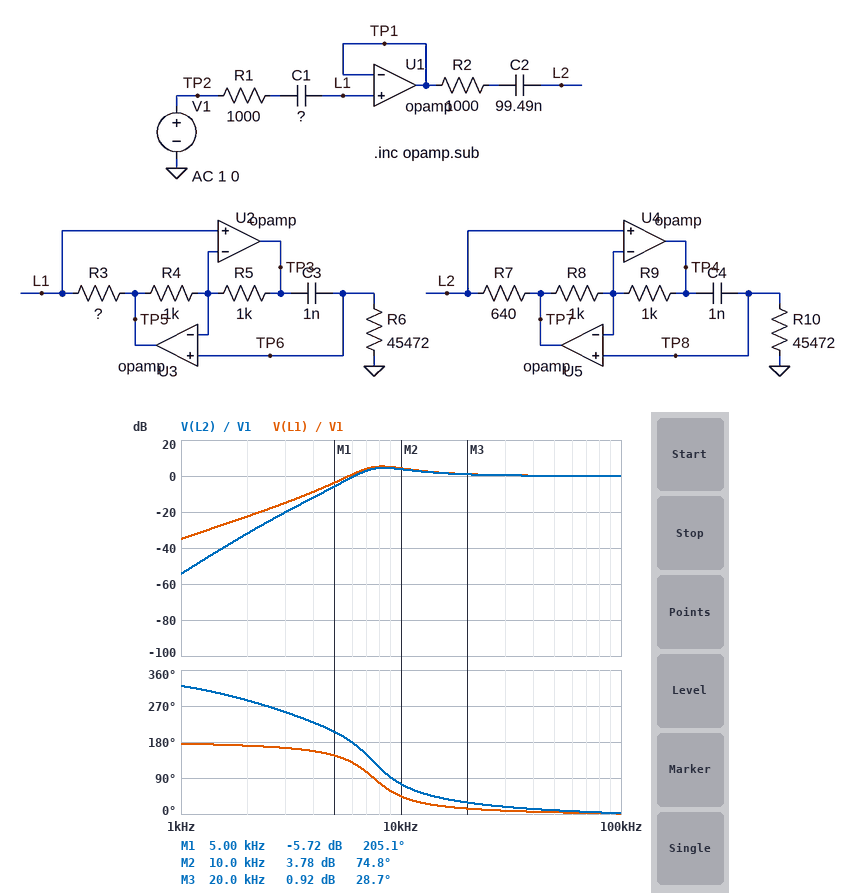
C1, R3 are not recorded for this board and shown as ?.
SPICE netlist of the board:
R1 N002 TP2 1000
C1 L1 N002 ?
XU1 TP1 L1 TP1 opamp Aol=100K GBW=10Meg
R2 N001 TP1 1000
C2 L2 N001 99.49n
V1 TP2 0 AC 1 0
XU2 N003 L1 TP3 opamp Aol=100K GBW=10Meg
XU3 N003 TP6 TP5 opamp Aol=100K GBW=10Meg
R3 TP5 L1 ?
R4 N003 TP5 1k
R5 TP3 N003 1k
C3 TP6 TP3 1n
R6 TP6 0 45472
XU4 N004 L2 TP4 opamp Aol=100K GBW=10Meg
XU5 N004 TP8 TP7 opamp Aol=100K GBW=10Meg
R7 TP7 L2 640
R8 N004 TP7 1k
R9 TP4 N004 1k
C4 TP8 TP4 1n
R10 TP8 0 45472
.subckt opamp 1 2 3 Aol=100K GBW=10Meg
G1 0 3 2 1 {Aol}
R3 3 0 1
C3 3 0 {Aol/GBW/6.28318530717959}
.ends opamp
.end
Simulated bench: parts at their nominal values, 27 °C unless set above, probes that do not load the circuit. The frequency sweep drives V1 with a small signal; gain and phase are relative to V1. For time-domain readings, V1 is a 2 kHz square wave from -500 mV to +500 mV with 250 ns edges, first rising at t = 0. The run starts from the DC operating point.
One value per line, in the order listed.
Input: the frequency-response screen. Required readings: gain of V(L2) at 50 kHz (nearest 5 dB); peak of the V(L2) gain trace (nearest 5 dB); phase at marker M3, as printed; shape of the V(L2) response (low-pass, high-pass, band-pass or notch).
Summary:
0 dB
5 dB
28.7 deg
high-pass
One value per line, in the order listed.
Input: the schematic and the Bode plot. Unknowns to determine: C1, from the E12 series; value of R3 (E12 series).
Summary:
12 nF
820 Ω
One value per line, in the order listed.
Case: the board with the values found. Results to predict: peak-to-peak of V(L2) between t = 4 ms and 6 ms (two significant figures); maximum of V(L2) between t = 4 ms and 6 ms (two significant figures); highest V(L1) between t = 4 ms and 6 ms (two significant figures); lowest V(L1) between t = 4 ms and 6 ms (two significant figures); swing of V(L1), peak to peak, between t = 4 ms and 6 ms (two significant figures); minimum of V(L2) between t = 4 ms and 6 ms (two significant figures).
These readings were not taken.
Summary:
1.9 V
940 mV
970 mV
-970 mV
1.9 V
-940 mV
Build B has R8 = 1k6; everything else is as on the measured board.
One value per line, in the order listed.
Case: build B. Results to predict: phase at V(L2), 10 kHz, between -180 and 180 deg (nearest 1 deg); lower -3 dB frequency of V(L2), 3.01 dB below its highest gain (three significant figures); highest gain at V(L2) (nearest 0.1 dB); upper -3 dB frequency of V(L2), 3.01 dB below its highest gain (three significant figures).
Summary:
89 deg
6.71 kHz
3.0 dB
200 kHz
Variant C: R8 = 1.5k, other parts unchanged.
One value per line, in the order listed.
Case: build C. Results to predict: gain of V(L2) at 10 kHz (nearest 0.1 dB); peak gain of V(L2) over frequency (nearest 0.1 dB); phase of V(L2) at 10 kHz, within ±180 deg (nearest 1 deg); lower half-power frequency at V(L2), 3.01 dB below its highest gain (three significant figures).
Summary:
2.8 dB
3.2 dB
87 deg
6.68 kHz
